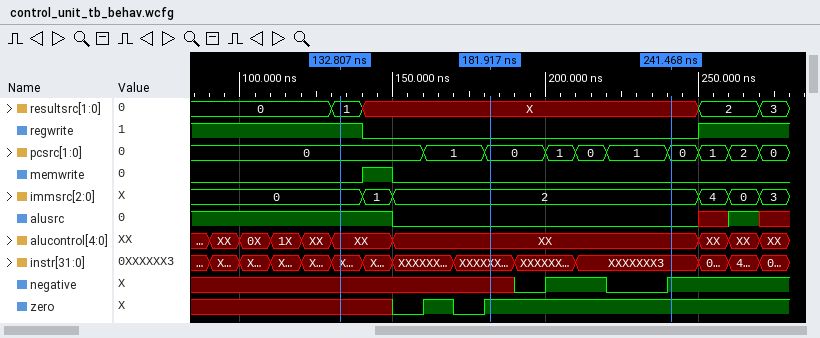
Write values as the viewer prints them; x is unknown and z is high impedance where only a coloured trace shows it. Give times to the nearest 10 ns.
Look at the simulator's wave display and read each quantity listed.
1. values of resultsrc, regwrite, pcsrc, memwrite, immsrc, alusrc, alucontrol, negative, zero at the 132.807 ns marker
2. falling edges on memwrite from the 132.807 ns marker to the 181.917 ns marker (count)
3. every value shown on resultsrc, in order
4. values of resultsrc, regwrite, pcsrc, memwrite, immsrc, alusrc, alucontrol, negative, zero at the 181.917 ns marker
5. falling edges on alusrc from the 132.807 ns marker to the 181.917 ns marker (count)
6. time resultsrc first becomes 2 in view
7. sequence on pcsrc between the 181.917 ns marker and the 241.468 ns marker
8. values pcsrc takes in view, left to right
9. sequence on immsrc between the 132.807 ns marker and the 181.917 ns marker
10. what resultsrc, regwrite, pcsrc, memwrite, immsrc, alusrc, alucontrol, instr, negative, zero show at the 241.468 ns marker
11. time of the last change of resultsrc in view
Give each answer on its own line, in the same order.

resultsrc=1, regwrite=1, pcsrc=0, memwrite=0, immsrc=0, alusrc=1, alucontrol=XX, negative=x, zero=x
1
0, 1, X, 2, 3
resultsrc=X, regwrite=0, pcsrc=0, memwrite=0, immsrc=2, alusrc=0, alucontrol=XX, negative=x, zero=1
1
250 ns
0, 1, 0, 1, 0
0, 1, 0, 1, 0, 1, 0, 1, 2, 0
0, 1, 2
resultsrc=X, regwrite=0, pcsrc=0, memwrite=0, immsrc=2, alusrc=0, alucontrol=XX, instr=XXXXXXX3, negative=1, zero=1
270 ns
